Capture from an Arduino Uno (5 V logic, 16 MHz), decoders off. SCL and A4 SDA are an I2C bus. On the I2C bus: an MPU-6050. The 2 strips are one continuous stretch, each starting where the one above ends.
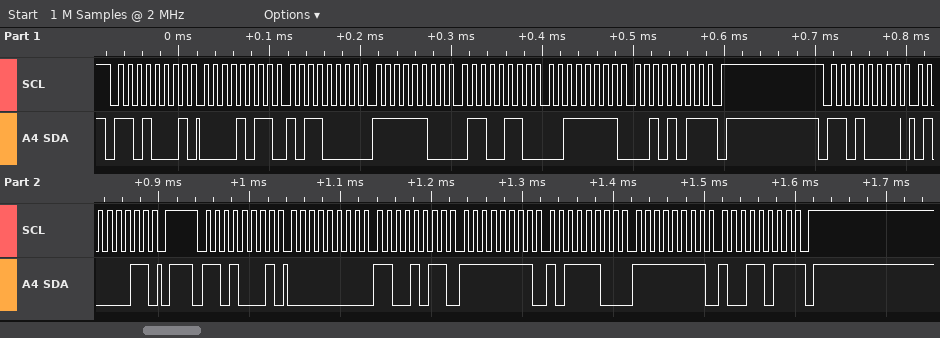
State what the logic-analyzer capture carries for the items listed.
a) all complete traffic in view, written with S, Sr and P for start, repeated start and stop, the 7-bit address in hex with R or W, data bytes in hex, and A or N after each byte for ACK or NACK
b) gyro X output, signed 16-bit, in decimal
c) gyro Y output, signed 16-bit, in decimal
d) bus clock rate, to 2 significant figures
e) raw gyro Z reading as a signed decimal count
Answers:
S 68R A 0B A B0 A FC A 66 A 3F A 2B N P S 68W A 43 A P S 68R A 00 A CB A FF A BC A FF A 9B N P
203
-68
100 kHz
-101
